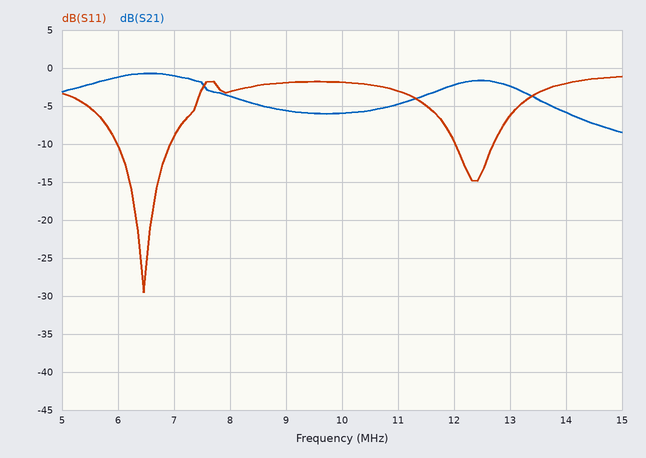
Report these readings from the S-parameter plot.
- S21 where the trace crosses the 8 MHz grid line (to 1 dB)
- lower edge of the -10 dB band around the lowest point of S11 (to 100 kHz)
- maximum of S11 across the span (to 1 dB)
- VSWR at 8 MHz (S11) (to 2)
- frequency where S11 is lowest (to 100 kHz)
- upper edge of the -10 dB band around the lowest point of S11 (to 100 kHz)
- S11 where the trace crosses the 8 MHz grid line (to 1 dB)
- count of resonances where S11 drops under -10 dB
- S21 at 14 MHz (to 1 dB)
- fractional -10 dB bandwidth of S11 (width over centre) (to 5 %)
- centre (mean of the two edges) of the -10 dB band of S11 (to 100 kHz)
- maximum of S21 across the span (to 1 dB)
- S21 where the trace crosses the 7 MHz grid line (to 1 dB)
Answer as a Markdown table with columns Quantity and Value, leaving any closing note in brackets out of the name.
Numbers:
| Quantity | Value |
|---|---|
| S21 where the trace crosses the 8 MHz grid line | -4 dB |
| lower edge of the -10 dB band around the lowest point of S11 | 6.0 MHz |
| maximum of S11 across the span | -1 dB |
| VSWR at 8 MHz (S11) | 6 |
| frequency where S11 is lowest | 6.5 MHz |
| upper edge of the -10 dB band around the lowest point of S11 | 6.9 MHz |
| S11 where the trace crosses the 8 MHz grid line | -3 dB |
| count of resonances where S11 drops under -10 dB | 2 |
| S21 at 14 MHz | -6 dB |
| fractional -10 dB bandwidth of S11 (width over centre) | 15 % |
| centre (mean of the two edges) of the -10 dB band of S11 | 6.5 MHz |
| maximum of S21 across the span | -1 dB |
| S21 where the trace crosses the 7 MHz grid line | -1 dB |
